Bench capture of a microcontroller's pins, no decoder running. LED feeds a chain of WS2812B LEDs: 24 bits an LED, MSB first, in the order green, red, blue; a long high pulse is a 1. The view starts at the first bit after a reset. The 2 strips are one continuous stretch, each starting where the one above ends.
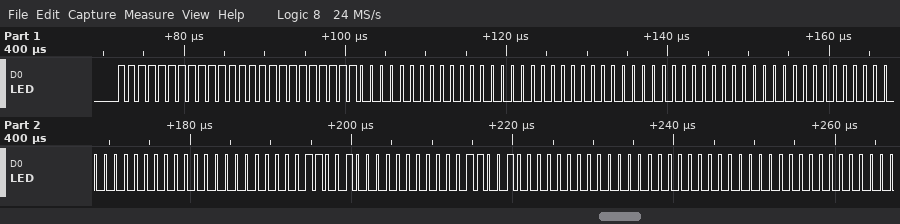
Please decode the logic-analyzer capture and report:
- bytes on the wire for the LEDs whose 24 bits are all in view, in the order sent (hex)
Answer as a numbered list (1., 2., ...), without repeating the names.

1. FF FF FF 00 00 00 00 00 00 00 00 00 32 00 32 00 00 00
